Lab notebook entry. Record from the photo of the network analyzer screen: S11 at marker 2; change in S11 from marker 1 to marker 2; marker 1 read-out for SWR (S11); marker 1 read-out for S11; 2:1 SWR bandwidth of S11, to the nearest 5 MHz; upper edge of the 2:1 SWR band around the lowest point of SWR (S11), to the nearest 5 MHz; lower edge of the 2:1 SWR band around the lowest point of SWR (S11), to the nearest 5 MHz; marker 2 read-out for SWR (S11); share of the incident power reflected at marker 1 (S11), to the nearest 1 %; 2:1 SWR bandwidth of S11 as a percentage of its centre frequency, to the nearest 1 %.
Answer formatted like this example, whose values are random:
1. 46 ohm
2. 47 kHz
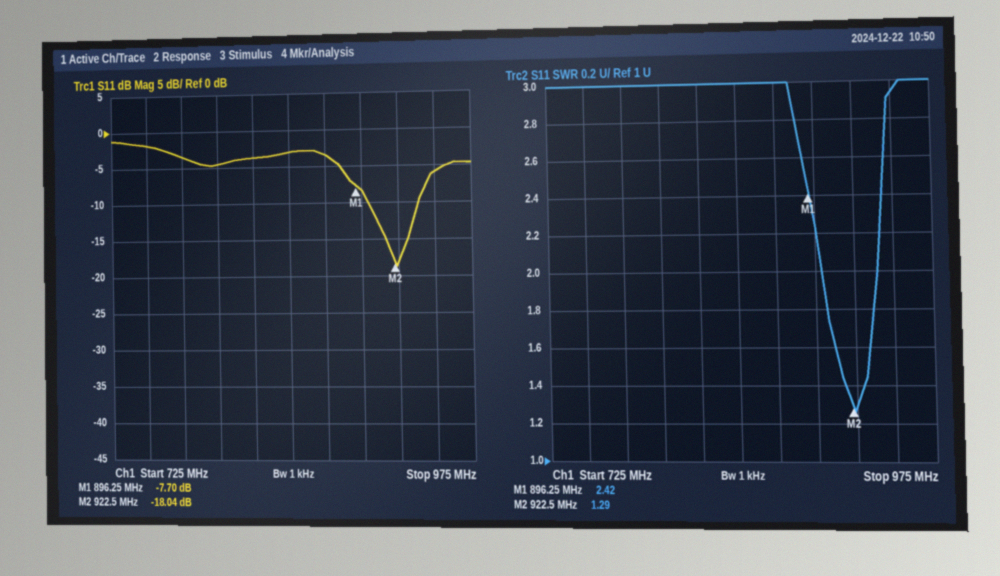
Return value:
1. -18.04 dB
2. -10.34 dB
3. 2.42
4. -7.70 dB
5. 35 MHz
6. 940 MHz
7. 905 MHz
8. 1.29
9. 17 %
10. 4 %
